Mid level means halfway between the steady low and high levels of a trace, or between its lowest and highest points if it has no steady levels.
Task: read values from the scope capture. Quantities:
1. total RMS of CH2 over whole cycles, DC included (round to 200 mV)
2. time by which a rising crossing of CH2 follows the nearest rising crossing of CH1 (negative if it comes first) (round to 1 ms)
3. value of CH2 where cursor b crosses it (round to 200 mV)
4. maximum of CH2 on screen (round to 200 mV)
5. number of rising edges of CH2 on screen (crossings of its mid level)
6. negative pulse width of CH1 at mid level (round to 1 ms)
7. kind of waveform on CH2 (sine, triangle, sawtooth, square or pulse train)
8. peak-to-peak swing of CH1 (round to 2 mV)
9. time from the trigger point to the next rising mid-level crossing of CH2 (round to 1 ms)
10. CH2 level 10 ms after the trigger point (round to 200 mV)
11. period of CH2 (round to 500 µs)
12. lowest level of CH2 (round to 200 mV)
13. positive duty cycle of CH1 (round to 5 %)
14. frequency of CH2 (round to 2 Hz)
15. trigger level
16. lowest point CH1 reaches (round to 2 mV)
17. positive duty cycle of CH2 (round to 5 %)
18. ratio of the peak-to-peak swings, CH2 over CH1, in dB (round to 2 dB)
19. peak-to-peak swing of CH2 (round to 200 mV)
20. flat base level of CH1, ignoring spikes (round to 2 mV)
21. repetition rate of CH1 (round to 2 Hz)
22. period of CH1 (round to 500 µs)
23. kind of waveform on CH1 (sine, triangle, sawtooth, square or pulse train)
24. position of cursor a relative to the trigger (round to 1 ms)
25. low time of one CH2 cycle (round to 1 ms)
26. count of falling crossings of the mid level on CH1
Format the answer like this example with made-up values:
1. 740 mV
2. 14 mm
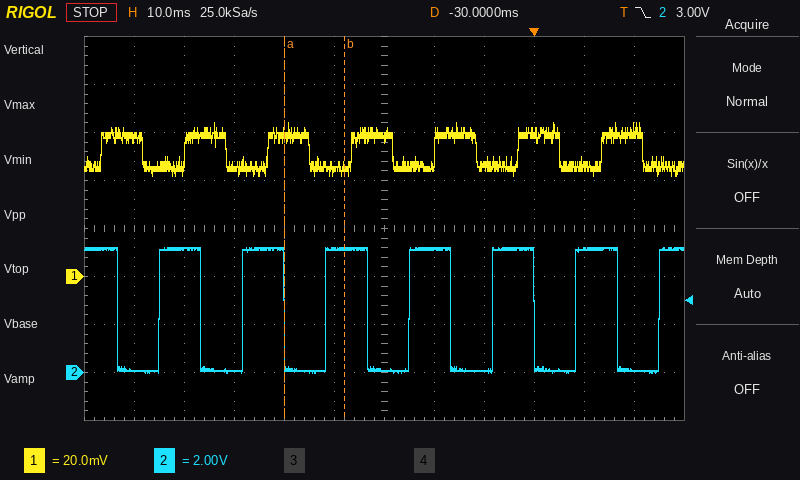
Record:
1. 3.6 V
2. -5 ms
3. 5.2 V
4. 5.2 V
5. 7
6. 8 ms
7. square
8. 22 mV
9. 8 ms
10. 5.2 V
11. 16.5 ms
12. 0.0 V
13. 50 %
14. 60 Hz
15. 3.00 V
16. 42 mV
17. 50 %
18. 48 dB
19. 5.2 V
20. 46 mV
21. 60 Hz
22. 16.5 ms
23. square
24. -50 ms
25. 8 ms
26. 7
